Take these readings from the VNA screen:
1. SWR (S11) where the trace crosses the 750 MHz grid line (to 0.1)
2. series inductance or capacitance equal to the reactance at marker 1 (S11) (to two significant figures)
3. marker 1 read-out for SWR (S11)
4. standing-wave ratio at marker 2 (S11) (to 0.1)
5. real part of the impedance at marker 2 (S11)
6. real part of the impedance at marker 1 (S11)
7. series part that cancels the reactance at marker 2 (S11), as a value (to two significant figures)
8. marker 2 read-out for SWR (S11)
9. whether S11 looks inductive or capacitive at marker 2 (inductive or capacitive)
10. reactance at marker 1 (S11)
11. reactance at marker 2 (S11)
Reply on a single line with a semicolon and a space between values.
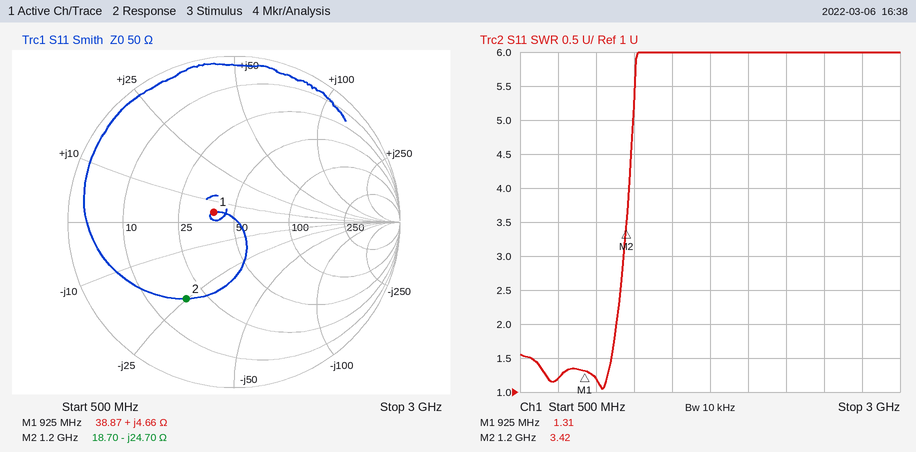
1.2; 800 pH; 1.31; 3.4; 18.70 Ω; 38.87 Ω; 3.3 nH; 3.42; capacitive; +4.66 Ω; -24.70 Ω
